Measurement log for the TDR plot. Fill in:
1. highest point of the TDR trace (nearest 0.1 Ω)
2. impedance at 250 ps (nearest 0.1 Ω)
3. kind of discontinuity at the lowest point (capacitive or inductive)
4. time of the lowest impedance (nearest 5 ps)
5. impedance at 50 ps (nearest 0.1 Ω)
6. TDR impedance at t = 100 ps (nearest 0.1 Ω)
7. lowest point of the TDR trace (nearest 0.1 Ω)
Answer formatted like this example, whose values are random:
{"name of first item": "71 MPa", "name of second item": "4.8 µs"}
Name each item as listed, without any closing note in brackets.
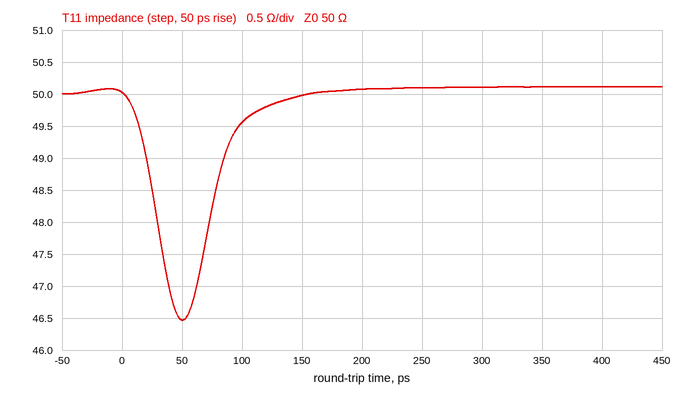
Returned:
{"highest point of the TDR trace": "50.1 Ω", "impedance at 250 ps": "50.1 Ω", "kind of discontinuity at the lowest point": "capacitive", "time of the lowest impedance": "50 ps", "impedance at 50 ps": "46.5 Ω", "TDR impedance at t = 100 ps": "49.6 Ω", "lowest point of the TDR trace": "46.5 Ω"}
